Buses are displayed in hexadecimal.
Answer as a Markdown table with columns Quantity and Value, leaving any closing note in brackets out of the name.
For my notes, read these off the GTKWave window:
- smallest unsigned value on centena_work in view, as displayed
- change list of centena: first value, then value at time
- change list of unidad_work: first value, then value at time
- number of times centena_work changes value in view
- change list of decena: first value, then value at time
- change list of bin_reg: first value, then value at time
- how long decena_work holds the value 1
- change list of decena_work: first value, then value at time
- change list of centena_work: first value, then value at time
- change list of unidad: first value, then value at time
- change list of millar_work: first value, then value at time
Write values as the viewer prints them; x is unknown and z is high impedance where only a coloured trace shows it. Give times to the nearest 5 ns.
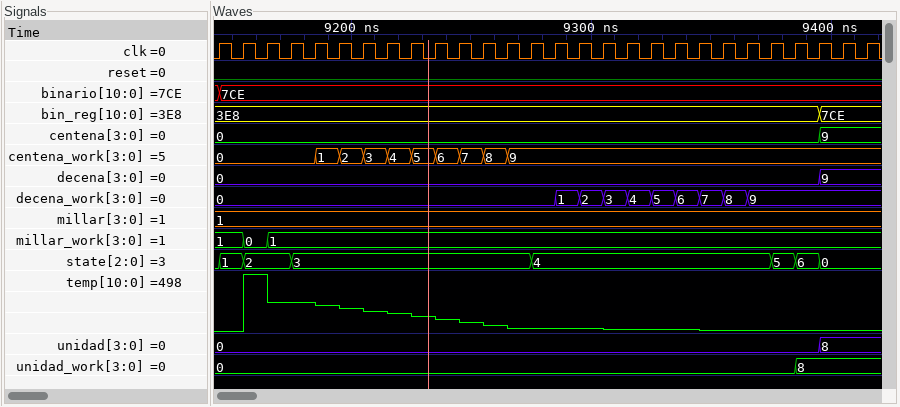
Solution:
| Quantity | Value |
|---|---|
| smallest unsigned value on centena_work in view, as displayed | 0 |
| change list of centena: first value, then value at time | 0, 9 at 9395 ns |
| change list of unidad_work: first value, then value at time | 0, 8 at 9385 ns |
| number of times centena_work changes value in view | 9 |
| change list of decena: first value, then value at time | 0, 9 at 9395 ns |
| change list of bin_reg: first value, then value at time | 3E8, 7CE at 9395 ns |
| how long decena_work holds the value 1 | 10 ns |
| change list of decena_work: first value, then value at time | 0, 1 at 9285 ns, 2 at 9295 ns, 3 at 9305 ns, 4 at 9315 ns, 5 at 9325 ns, 6 at 9335 ns, 7 at 9345 ns, 8 at 9355 ns, 9 at 9365 ns |
| change list of centena_work: first value, then value at time | 0, 1 at 9185 ns, 2 at 9195 ns, 3 at 9205 ns, 4 at 9215 ns, 5 at 9225 ns, 6 at 9235 ns, 7 at 9245 ns, 8 at 9255 ns, 9 at 9265 ns |
| change list of unidad: first value, then value at time | 0, 8 at 9395 ns |
| change list of millar_work: first value, then value at time | 1, 0 at 9155 ns, 1 at 9165 ns |
